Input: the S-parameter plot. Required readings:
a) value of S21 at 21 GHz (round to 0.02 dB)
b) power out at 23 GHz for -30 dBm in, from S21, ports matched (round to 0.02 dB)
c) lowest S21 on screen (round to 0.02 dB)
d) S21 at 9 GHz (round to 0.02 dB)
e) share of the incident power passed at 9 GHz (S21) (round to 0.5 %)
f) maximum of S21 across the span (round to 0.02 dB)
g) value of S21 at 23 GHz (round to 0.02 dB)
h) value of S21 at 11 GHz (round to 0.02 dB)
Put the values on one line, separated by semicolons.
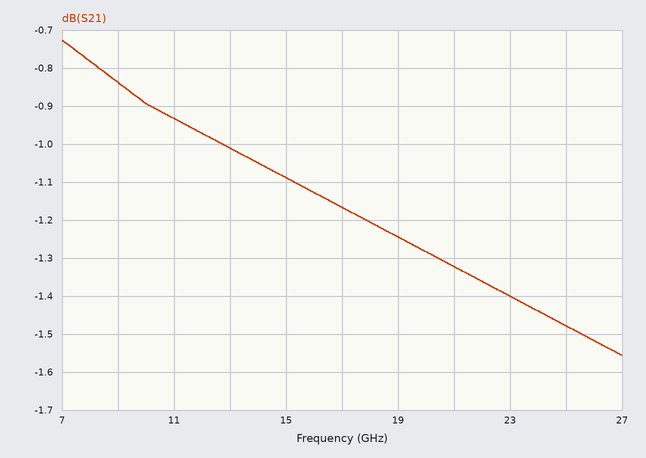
-1.32 dB; -31.40 dBm; -1.56 dB; -0.84 dB; 82.5 %; -0.72 dB; -1.40 dB; -0.94 dB
